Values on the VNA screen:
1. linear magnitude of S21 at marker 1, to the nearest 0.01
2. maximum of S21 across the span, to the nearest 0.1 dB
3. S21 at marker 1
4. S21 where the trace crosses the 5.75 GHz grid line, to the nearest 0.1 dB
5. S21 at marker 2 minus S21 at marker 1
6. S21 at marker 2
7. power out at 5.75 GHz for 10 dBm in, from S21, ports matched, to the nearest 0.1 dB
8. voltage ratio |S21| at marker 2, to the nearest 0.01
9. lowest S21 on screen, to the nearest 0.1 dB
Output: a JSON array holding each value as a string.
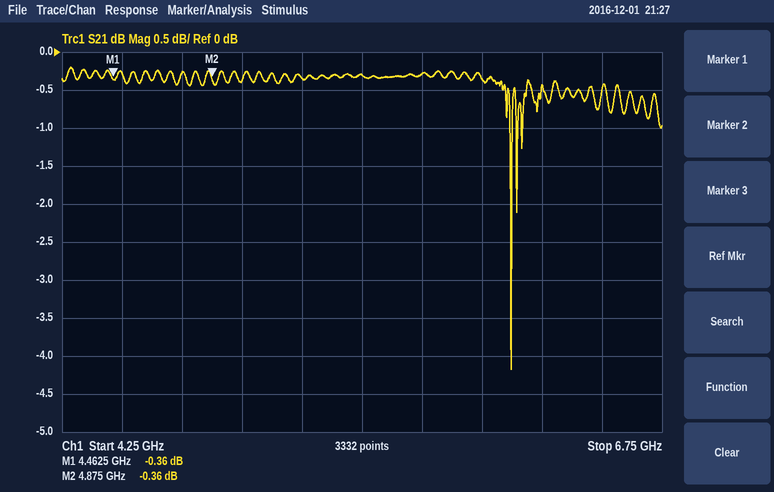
["0.96", "-0.2 dB", "-0.36 dB", "-0.3 dB", "0.00 dB", "-0.36 dB", "9.7 dBm", "0.96", "-4.2 dB"]
